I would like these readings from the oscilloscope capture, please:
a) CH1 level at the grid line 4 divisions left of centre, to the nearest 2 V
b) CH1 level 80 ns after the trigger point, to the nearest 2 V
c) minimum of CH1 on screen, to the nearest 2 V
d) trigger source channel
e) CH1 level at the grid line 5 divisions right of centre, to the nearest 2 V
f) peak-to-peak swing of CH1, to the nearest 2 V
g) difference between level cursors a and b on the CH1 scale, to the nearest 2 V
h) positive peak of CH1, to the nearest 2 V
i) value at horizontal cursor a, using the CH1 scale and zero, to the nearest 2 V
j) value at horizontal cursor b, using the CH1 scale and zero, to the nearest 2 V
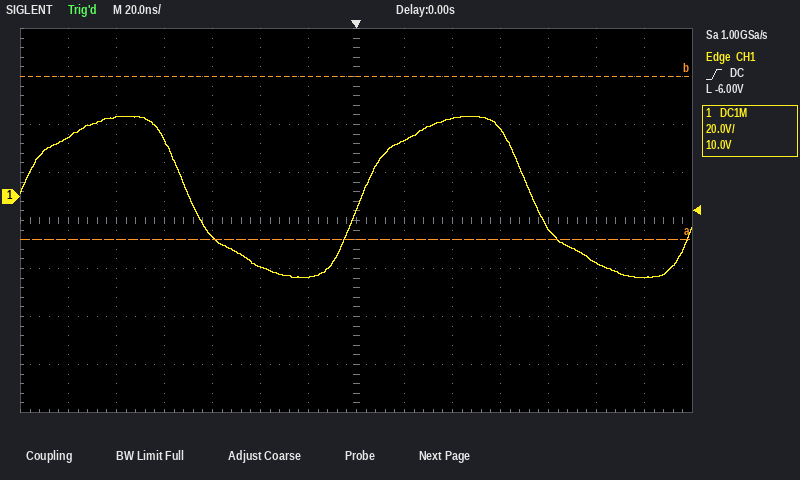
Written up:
24 V
-14 V
-34 V
CH1
-28 V
68 V
68 V
34 V
-18 V
50 V
